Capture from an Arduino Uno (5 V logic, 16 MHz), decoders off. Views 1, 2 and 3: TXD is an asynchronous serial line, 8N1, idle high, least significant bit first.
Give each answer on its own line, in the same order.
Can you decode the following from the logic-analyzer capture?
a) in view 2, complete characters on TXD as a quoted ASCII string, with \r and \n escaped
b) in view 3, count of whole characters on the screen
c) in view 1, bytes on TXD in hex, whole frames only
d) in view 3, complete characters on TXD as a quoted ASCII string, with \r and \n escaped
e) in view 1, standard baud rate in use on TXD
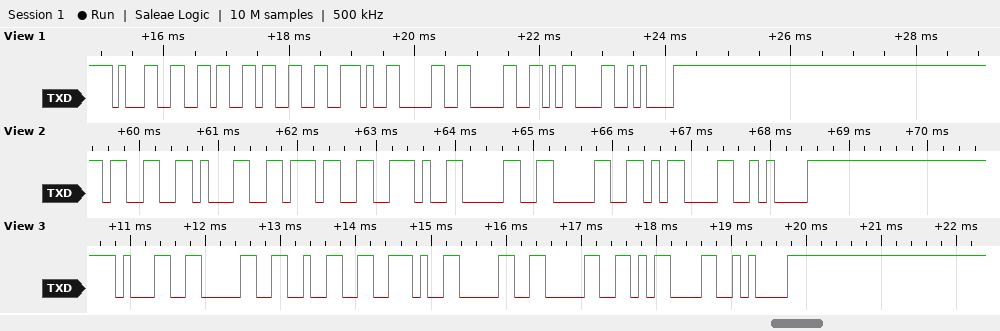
"317.00\r\n"
8
0x31 0x36 0x33 0x2E 0x30 0x30 0x0D 0x0A
"102.00\r\n"
9600 baud
